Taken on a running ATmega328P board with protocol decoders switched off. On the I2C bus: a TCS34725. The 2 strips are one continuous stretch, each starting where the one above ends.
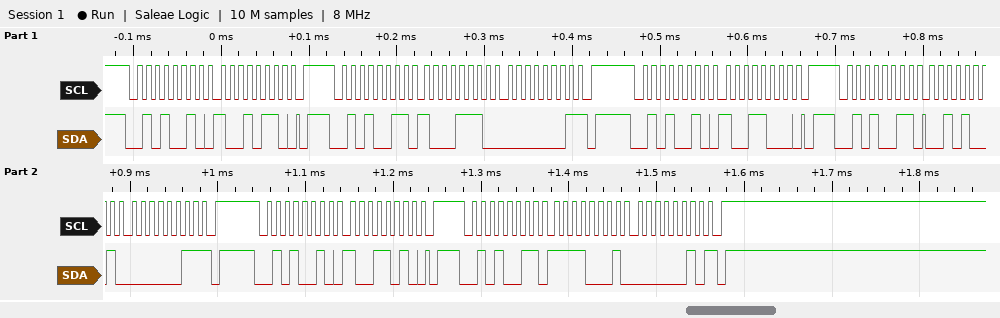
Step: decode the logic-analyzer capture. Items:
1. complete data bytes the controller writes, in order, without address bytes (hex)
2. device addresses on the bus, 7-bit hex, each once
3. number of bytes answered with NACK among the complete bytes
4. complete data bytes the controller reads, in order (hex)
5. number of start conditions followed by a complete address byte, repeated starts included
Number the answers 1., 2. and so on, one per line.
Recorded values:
1. 96 98 9A
2. 0x29
3. 3
4. 8E 01 29 03 F1 02
5. 6
